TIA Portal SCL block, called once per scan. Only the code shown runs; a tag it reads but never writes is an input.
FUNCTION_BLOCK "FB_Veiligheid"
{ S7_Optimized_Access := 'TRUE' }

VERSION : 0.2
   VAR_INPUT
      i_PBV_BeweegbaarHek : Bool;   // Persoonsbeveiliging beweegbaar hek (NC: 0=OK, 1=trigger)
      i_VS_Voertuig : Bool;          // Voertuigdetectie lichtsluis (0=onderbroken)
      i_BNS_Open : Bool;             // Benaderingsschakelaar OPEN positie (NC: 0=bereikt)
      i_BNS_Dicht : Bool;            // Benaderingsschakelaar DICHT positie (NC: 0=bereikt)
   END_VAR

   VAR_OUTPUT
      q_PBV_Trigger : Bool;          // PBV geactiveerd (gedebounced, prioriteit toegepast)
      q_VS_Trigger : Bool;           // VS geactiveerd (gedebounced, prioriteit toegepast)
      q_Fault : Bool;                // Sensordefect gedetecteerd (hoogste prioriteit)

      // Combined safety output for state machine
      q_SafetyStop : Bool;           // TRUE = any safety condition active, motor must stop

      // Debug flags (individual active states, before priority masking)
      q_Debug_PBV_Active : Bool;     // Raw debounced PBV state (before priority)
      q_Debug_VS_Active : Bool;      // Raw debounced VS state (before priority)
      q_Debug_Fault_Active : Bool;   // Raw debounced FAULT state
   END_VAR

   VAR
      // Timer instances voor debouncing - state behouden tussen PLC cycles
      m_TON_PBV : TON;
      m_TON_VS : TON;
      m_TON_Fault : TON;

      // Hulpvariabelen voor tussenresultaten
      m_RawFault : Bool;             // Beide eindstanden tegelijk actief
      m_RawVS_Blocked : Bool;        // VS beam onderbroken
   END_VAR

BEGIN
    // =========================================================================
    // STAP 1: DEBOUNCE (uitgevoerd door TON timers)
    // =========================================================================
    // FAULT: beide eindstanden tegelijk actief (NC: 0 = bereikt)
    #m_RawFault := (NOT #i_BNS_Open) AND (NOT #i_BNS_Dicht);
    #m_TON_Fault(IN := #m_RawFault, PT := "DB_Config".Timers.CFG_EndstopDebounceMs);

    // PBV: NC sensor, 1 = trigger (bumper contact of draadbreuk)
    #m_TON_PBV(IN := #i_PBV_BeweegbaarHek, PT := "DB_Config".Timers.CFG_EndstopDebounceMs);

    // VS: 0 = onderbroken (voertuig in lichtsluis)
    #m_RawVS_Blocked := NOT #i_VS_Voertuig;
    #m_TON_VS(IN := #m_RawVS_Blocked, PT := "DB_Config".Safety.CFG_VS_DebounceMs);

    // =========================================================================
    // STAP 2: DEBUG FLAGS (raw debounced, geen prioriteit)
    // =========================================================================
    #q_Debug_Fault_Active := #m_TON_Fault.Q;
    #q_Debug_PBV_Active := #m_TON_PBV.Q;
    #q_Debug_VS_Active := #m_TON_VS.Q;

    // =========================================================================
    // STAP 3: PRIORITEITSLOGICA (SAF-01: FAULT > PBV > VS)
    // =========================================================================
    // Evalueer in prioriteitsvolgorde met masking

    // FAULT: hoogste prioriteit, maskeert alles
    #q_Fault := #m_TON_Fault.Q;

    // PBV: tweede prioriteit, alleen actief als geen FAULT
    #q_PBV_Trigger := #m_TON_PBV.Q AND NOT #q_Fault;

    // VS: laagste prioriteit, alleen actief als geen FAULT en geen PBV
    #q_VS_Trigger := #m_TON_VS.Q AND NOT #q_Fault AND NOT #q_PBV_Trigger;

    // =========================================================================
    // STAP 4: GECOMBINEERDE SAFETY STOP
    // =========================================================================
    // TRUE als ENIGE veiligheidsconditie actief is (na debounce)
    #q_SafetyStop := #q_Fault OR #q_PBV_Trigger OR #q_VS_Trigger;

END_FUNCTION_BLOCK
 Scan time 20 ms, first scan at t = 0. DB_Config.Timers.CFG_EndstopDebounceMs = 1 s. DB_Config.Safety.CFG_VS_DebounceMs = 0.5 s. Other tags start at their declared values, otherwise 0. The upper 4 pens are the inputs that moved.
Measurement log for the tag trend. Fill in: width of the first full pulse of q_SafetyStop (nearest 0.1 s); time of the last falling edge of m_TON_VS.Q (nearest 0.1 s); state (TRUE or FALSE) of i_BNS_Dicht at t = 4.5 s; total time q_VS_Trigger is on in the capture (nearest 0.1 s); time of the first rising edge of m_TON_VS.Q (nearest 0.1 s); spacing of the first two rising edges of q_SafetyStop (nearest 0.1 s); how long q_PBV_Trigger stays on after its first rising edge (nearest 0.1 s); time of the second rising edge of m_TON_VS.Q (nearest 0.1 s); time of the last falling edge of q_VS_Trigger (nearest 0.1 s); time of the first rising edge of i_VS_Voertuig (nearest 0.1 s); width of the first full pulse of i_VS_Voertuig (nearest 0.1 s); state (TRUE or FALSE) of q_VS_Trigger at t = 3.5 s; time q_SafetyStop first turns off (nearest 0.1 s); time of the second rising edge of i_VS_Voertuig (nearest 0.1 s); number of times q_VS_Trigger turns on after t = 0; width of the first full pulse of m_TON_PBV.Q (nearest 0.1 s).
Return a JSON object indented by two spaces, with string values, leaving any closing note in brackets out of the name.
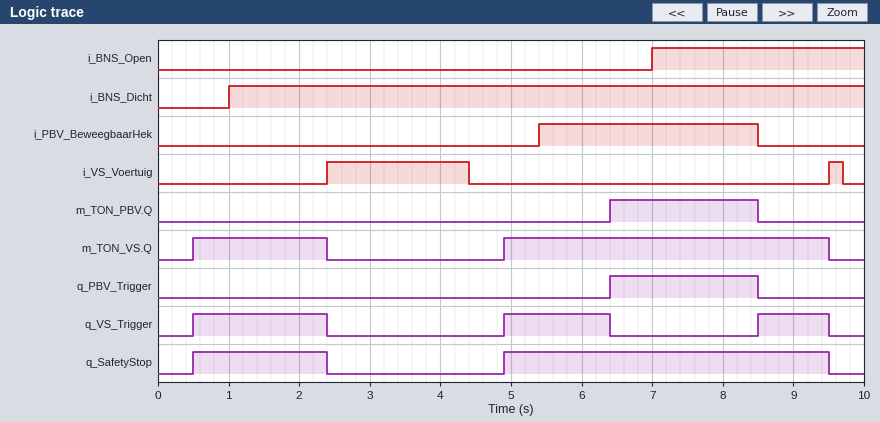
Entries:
{
  "width of the first full pulse of q_SafetyStop": "1.9 s",
  "time of the last falling edge of m_TON_VS.Q": "9.5 s",
  "state (TRUE or FALSE) of i_BNS_Dicht at t = 4.5 s": "TRUE",
  "total time q_VS_Trigger is on in the capture": "4.4 s",
  "time of the first rising edge of m_TON_VS.Q": "0.5 s",
  "spacing of the first two rising edges of q_SafetyStop": "4.4 s",
  "how long q_PBV_Trigger stays on after its first rising edge": "2.1 s",
  "time of the second rising edge of m_TON_VS.Q": "4.9 s",
  "time of the last falling edge of q_VS_Trigger": "9.5 s",
  "time of the first rising edge of i_VS_Voertuig": "2.4 s",
  "width of the first full pulse of i_VS_Voertuig": "2.0 s",
  "state (TRUE or FALSE) of q_VS_Trigger at t = 3.5 s": "FALSE",
  "time q_SafetyStop first turns off": "2.4 s",
  "time of the second rising edge of i_VS_Voertuig": "9.5 s",
  "number of times q_VS_Trigger turns on after t = 0": "3",
  "width of the first full pulse of m_TON_PBV.Q": "2.1 s"
}
